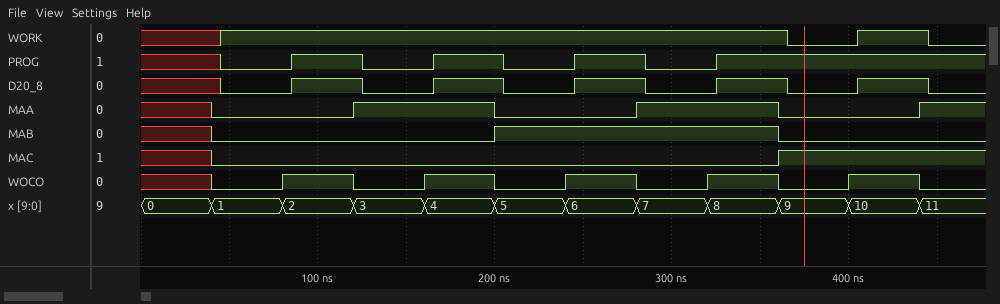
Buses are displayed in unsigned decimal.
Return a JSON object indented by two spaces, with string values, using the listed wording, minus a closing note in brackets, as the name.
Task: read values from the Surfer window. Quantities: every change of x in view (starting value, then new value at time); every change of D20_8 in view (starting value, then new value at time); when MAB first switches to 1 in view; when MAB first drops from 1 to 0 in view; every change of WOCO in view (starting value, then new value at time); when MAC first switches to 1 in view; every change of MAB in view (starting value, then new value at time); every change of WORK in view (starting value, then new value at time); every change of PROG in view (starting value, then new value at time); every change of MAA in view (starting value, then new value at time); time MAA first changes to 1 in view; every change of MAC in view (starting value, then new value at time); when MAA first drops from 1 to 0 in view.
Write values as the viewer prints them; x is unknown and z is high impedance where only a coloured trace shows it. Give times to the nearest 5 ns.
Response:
{
  "every change of x in view": "0, 1 at 40 ns, 2 at 80 ns, 3 at 120 ns, 4 at 160 ns, 5 at 200 ns, 6 at 240 ns, 7 at 280 ns, 8 at 320 ns, 9 at 360 ns, 10 at 400 ns, 11 at 440 ns",
  "every change of D20_8 in view": "x, 0 at 45 ns, 1 at 85 ns, 0 at 125 ns, 1 at 165 ns, 0 at 205 ns, 1 at 245 ns, 0 at 285 ns, 1 at 325 ns, 0 at 365 ns, 1 at 405 ns, 0 at 445 ns",
  "when MAB first switches to 1 in view": "200 ns",
  "when MAB first drops from 1 to 0 in view": "360 ns",
  "every change of WOCO in view": "x, 0 at 40 ns, 1 at 80 ns, 0 at 120 ns, 1 at 160 ns, 0 at 200 ns, 1 at 240 ns, 0 at 280 ns, 1 at 320 ns, 0 at 360 ns, 1 at 400 ns, 0 at 440 ns",
  "when MAC first switches to 1 in view": "360 ns",
  "every change of MAB in view": "x, 0 at 40 ns, 1 at 200 ns, 0 at 360 ns",
  "every change of WORK in view": "x, 1 at 45 ns, 0 at 365 ns, 1 at 405 ns, 0 at 445 ns",
  "every change of PROG in view": "x, 0 at 45 ns, 1 at 85 ns, 0 at 125 ns, 1 at 165 ns, 0 at 205 ns, 1 at 245 ns, 0 at 285 ns, 1 at 325 ns",
  "every change of MAA in view": "x, 0 at 40 ns, 1 at 120 ns, 0 at 200 ns, 1 at 280 ns, 0 at 360 ns, 1 at 440 ns",
  "time MAA first changes to 1 in view": "120 ns",
  "every change of MAC in view": "x, 0 at 40 ns, 1 at 360 ns",
  "when MAA first drops from 1 to 0 in view": "200 ns"
}
